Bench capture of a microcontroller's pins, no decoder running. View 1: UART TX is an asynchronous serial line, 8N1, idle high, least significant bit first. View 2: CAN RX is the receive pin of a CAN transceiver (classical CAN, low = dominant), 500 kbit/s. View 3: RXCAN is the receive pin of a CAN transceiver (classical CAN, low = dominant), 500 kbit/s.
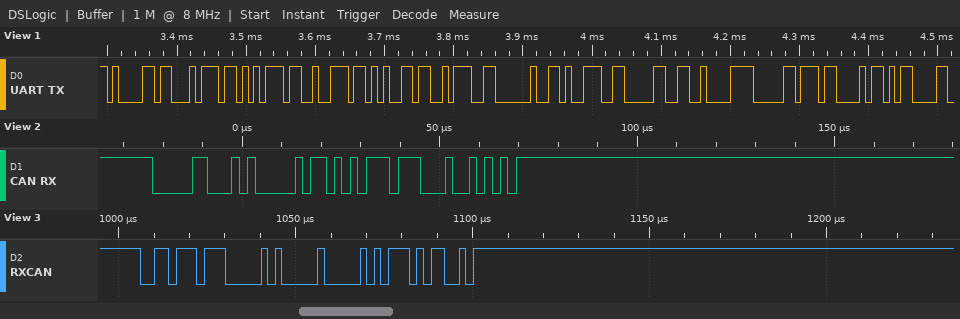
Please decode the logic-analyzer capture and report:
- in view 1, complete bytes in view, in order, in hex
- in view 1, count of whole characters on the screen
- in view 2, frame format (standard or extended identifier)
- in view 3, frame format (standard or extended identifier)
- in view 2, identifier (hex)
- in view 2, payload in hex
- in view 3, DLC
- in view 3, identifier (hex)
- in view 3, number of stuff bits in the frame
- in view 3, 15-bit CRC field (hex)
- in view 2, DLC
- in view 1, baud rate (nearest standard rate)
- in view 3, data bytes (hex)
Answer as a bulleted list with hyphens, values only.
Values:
- 61 74 75 72 65 3A 20 39 30 C2 B0 43 0D
- 13
- standard
- standard
- 0x045
- AB
- 1
- 0x377
- 3
- 0x0BAC
- 1
- 115200 baud
- 00
